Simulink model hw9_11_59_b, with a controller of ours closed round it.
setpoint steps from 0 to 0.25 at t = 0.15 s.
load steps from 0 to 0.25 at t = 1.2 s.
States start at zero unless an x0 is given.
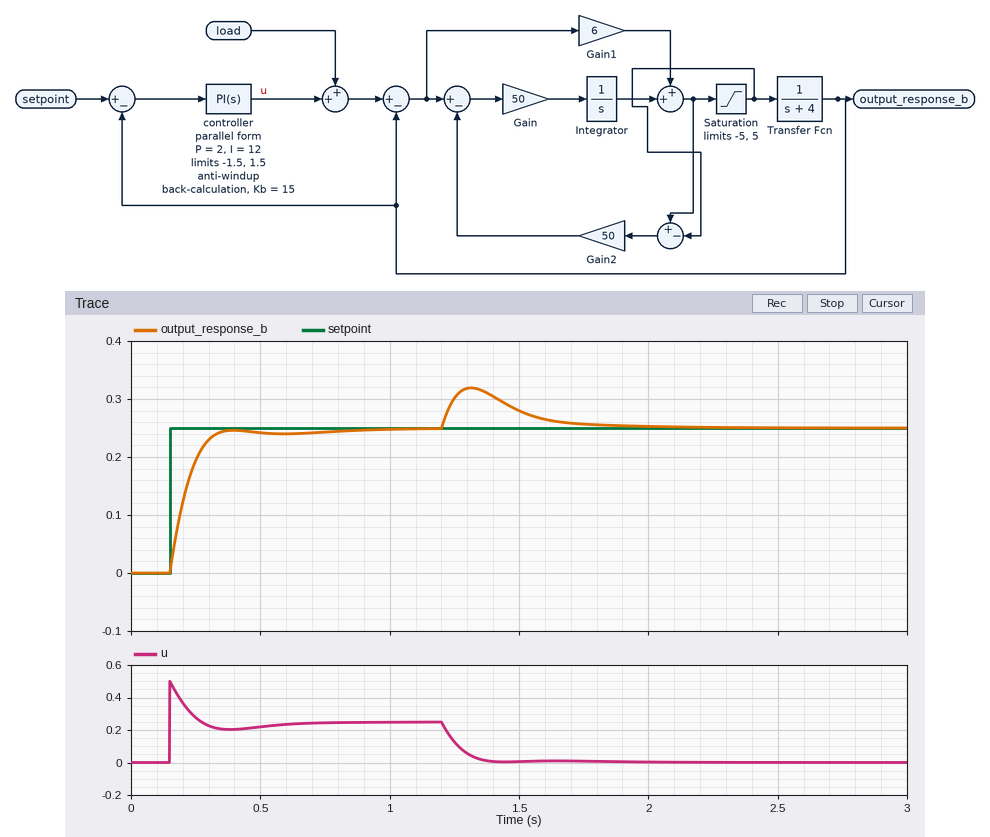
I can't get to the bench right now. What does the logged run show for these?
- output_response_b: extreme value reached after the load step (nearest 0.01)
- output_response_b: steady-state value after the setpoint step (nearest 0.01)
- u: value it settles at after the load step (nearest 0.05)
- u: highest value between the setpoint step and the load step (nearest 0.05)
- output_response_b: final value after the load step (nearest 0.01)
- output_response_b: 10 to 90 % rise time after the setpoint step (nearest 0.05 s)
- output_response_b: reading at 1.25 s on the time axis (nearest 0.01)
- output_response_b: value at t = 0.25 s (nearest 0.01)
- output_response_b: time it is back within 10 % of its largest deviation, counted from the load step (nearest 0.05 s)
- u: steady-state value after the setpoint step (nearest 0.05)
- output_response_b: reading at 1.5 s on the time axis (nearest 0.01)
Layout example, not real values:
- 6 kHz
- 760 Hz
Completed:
- 0.32
- 0.25
- 0.00
- 0.50
- 0.25
- 0.15 s
- 0.30
- 0.19
- 0.55 s
- 0.25
- 0.28
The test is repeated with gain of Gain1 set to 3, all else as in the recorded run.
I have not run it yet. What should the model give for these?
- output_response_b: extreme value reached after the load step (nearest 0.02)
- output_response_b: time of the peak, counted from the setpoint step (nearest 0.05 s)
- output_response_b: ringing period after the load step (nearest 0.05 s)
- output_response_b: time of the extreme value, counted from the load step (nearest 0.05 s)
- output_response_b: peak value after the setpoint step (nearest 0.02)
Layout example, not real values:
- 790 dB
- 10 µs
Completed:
- 0.32
- 0.25 s
- 0.55 s
- 0.15 s
- 0.28
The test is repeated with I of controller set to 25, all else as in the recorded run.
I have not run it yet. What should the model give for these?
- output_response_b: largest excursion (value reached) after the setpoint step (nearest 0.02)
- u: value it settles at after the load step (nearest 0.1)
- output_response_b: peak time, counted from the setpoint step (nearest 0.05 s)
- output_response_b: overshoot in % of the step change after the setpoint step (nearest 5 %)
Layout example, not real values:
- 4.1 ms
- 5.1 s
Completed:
- 0.28
- 0.0
- 0.20 s
- 10 %
